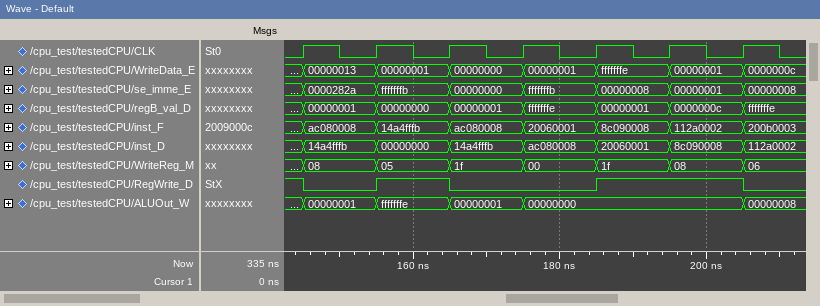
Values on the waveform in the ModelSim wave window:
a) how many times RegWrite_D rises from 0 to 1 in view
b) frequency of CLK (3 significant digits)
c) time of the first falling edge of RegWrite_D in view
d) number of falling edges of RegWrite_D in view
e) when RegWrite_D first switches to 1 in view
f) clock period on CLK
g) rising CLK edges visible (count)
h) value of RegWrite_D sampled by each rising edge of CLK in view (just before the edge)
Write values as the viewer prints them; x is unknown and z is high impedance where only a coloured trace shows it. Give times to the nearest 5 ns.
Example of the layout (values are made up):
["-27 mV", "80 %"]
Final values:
["2", "100 MHz", "145 ns", "3", "155 ns", "10 ns", "7", "1 0 1 0 0 1 1"]
